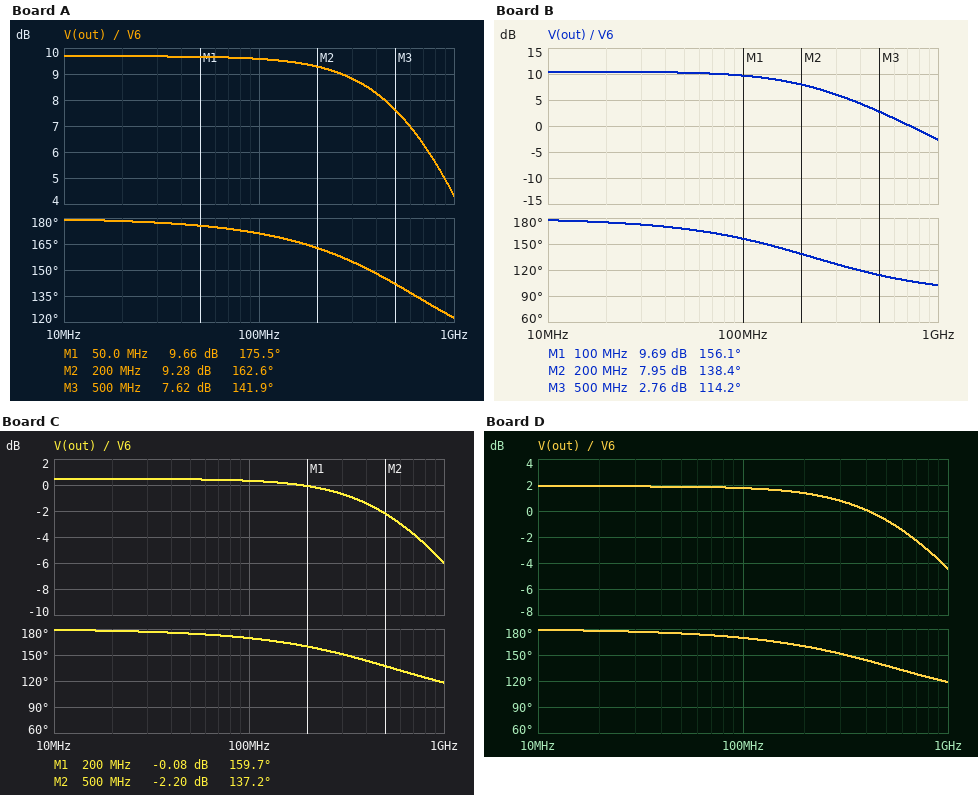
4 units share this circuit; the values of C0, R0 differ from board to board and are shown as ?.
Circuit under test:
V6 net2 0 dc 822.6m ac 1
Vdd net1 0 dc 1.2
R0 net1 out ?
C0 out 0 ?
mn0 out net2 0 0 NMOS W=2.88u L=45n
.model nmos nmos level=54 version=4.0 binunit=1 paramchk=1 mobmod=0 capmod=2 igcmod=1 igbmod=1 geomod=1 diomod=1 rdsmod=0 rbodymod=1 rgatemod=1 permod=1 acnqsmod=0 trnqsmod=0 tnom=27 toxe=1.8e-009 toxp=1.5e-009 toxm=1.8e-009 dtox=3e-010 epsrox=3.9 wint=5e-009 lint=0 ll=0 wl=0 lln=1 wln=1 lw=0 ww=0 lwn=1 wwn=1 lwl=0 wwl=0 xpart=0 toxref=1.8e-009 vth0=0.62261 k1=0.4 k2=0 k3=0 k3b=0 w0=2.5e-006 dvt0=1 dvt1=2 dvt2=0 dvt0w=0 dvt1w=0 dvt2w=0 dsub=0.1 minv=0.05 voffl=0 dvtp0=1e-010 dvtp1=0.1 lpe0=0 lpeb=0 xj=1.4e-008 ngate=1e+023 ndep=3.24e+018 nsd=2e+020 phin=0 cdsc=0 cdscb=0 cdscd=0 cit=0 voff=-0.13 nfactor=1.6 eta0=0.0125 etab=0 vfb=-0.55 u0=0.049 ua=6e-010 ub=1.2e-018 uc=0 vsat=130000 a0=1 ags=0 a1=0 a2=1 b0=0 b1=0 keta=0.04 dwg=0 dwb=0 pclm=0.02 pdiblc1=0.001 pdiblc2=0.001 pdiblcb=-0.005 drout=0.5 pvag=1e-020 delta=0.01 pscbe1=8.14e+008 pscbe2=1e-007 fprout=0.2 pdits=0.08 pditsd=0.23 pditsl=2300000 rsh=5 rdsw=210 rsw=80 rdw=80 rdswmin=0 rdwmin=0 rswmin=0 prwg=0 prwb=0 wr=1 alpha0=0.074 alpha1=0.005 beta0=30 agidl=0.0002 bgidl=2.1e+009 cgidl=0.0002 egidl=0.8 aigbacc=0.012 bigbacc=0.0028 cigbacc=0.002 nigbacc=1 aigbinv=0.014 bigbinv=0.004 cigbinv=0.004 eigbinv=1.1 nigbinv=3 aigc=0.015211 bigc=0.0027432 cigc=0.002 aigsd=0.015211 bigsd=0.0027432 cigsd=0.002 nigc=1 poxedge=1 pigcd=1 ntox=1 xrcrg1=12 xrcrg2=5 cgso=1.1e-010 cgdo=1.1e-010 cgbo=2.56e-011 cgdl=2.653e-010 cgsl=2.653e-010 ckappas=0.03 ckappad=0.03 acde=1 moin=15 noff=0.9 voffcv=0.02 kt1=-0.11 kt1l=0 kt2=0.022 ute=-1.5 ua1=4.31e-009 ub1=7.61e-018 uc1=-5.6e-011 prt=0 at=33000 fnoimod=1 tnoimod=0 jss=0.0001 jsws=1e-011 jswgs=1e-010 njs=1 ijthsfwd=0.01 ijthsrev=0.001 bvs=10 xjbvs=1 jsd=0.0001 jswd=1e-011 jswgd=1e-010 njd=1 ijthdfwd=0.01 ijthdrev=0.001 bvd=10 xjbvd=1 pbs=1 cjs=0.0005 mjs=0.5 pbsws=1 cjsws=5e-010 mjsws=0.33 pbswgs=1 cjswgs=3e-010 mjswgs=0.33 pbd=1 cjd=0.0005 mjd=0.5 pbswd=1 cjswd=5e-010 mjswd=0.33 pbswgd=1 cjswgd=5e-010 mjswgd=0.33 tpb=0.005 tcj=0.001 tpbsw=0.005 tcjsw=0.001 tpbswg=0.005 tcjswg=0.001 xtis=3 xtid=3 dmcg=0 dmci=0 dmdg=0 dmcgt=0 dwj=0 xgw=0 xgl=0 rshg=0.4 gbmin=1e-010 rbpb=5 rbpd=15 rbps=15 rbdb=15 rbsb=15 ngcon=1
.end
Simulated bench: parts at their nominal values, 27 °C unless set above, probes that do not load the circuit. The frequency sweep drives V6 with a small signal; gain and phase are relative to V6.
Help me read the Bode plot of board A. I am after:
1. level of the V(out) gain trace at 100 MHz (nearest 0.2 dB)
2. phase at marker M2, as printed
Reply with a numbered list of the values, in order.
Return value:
1. 9.6 dB
2. 162.6 deg
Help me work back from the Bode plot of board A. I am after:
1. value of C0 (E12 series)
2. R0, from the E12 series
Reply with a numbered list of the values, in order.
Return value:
1. 220 fF
2. 1.5 kΩ
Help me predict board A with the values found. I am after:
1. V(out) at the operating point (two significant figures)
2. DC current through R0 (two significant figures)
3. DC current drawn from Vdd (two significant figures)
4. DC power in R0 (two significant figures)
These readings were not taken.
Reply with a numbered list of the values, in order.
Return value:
1. 480 mV
2. 480 µA
3. 480 µA
4. 340 µW
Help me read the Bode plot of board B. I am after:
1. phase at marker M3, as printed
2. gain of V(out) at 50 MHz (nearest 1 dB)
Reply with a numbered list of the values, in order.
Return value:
1. 114.2 deg
2. 10 dB
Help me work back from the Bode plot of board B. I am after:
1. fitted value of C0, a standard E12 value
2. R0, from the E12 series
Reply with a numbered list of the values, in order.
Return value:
1. 560 fF
2. 1.8 kΩ
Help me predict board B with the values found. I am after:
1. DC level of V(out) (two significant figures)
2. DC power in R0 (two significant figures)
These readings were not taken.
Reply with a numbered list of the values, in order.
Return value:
1. 380 mV
2. 370 µW
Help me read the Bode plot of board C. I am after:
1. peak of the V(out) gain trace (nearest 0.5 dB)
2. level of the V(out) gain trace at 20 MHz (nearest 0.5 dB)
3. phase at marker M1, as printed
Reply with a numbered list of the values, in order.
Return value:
1. 0.5 dB
2. 0.5 dB
3. 159.7 deg
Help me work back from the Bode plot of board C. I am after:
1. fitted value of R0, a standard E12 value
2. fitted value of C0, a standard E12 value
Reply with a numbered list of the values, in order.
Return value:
1. 390 Ω
2. 820 fF
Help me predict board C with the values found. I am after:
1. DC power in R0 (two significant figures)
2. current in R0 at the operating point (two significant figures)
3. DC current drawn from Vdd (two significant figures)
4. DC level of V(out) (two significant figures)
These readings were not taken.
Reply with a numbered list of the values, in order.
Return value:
1. 140 µW
2. 590 µA
3. 590 µA
4. 970 mV
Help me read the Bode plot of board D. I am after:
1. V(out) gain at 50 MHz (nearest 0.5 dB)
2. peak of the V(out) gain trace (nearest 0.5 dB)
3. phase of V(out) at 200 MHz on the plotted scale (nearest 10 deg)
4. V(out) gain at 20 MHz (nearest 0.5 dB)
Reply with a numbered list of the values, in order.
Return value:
1. 2.0 dB
2. 2.0 dB
3. 160 deg
4. 2.0 dB
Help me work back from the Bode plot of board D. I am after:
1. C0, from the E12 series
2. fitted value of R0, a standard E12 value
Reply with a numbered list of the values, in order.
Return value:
1. 680 fF
2. 470 Ω
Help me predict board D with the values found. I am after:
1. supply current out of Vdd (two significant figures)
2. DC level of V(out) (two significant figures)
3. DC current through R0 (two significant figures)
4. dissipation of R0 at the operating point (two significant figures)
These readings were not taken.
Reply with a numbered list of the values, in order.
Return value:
1. 580 µA
2. 930 mV
3. 580 µA
4. 160 µW
